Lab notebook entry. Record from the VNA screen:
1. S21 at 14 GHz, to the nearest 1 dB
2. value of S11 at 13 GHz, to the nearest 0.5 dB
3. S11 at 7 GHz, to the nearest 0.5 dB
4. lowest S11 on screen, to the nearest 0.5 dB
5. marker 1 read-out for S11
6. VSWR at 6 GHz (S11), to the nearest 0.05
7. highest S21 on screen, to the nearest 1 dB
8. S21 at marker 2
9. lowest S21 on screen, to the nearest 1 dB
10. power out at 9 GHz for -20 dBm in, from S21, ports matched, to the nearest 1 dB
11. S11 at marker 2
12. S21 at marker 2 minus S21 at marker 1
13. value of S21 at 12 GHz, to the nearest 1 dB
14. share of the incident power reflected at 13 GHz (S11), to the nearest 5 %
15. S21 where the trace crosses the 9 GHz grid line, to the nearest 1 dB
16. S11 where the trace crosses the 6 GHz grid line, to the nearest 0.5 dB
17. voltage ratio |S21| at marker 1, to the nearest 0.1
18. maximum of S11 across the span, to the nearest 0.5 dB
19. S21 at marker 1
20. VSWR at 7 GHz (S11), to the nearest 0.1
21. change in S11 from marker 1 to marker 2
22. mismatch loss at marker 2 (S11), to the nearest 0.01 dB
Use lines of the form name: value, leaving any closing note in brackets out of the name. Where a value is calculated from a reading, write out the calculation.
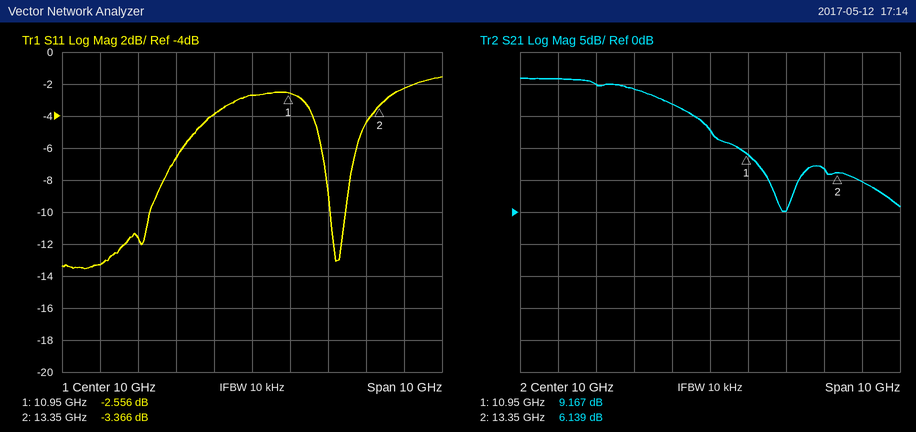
S21 at 14 GHz, to the nearest 1 dB: 5 dB
value of S11 at 13 GHz, to the nearest 0.5 dB: -4.5 dB
S11 at 7 GHz, to the nearest 0.5 dB: -11.5 dB
lowest S11 on screen, to the nearest 0.5 dB: -13.5 dB
marker 1 read-out for S11: -2.556 dB
VSWR at 6 GHz (S11), to the nearest 0.05: |Γ| = 10^(-13.5/20) = 0.2113; VSWR = (1 + 0.2113)/(1 − 0.2113) ≈ 1.54, so 1.55 to the nearest 0.05
highest S21 on screen, to the nearest 1 dB: 21 dB
S21 at marker 2: 6.139 dB
lowest S21 on screen, to the nearest 1 dB: 0 dB
power out at 9 GHz for -20 dBm in, from S21, ports matched, to the nearest 1 dB: -20 dBm + (17 dB) = -3 dBm
S11 at marker 2: -3.366 dB
S21 at marker 2 minus S21 at marker 1: 6.139 − (9.167) = -3.028 dB
value of S21 at 12 GHz, to the nearest 1 dB: 0 dB
share of the incident power reflected at 13 GHz (S11), to the nearest 5 %: 10^(-4.5/10) ≈ 35 %
S21 where the trace crosses the 9 GHz grid line, to the nearest 1 dB: 17 dB
S11 where the trace crosses the 6 GHz grid line, to the nearest 0.5 dB: -13.5 dB
voltage ratio |S21| at marker 1, to the nearest 0.1: 10^(9.167/20) ≈ 2.9
maximum of S11 across the span, to the nearest 0.5 dB: -1.5 dB
S21 at marker 1: 9.167 dB
VSWR at 7 GHz (S11), to the nearest 0.1: |Γ| = 10^(-11.5/20) = 0.2661; VSWR = (1 + 0.2661)/(1 − 0.2661) ≈ 1.7
change in S11 from marker 1 to marker 2: -3.366 − (-2.556) = -0.810 dB
mismatch loss at marker 2 (S11), to the nearest 0.01 dB: −10 log10(1 − 10^(-3.366/10)) ≈ 2.68 dB
